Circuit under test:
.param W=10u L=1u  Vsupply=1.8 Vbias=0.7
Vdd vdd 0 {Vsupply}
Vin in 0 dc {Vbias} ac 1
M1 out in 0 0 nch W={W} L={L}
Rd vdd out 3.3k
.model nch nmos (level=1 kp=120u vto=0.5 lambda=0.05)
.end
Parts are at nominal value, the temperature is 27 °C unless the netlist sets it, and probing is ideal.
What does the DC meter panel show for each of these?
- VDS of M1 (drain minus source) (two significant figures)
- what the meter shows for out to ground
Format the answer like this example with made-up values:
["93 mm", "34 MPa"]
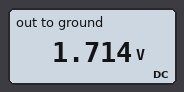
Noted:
["1.7 V", "1.714 V"]
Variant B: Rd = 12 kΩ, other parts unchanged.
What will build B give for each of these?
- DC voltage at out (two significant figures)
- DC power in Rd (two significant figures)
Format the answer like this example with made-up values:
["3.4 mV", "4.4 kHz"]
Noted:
["1.5 V", "8.0 µW"]
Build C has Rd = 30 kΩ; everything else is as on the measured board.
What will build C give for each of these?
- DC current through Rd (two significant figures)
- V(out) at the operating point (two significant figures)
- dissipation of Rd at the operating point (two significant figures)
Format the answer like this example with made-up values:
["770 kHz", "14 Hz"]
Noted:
["25 µA", "1.0 V", "19 µW"]
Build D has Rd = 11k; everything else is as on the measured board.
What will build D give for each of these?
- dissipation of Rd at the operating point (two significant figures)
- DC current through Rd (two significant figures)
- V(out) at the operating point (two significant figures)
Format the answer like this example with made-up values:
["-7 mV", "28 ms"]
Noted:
["7.3 µW", "26 µA", "1.5 V"]
